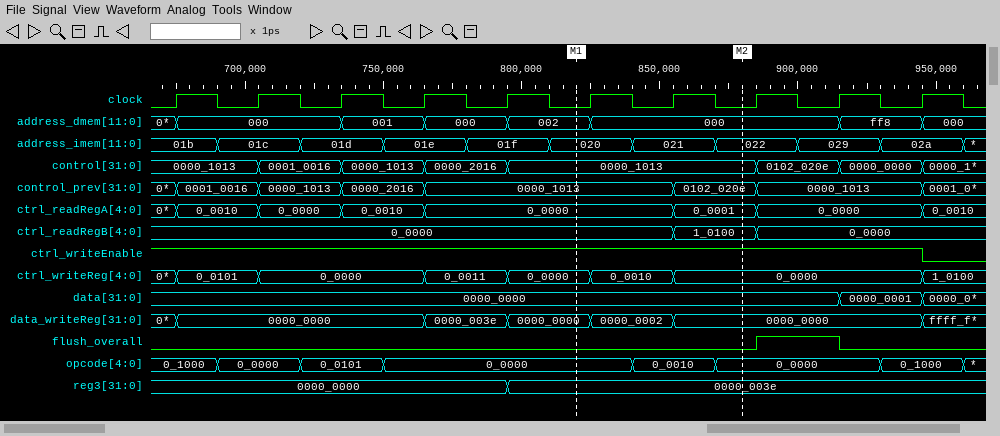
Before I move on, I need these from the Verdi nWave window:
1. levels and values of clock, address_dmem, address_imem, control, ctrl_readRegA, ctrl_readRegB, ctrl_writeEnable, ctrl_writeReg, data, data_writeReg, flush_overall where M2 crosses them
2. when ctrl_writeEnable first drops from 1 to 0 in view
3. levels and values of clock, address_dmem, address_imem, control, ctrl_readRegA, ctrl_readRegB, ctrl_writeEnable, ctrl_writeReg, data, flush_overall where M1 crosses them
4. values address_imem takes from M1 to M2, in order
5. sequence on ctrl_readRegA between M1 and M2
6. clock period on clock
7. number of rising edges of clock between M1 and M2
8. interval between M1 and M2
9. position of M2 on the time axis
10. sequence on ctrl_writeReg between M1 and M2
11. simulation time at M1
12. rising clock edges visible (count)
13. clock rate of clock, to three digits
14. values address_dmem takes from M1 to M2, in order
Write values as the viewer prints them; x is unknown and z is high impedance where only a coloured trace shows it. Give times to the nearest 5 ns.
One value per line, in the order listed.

clock=0, address_dmem=000, address_imem=022, control=0000_1013, ctrl_readRegA=0_0001, ctrl_readRegB=1_0100, ctrl_writeEnable=1, ctrl_writeReg=0_0000, data=0000_0000, data_writeReg=0000_0000, flush_overall=0
945 ns
clock=0, address_dmem=002, address_imem=020, control=0000_1013, ctrl_readRegA=0_0000, ctrl_readRegB=0_0000, ctrl_writeEnable=1, ctrl_writeReg=0_0000, data=0000_0000, flush_overall=0
020, 021, 022
0_0000, 0_0001
30 ns
2
60 ns
880 ns
0_0000, 0_0010, 0_0000
820 ns
10
33.3 MHz
002, 000
